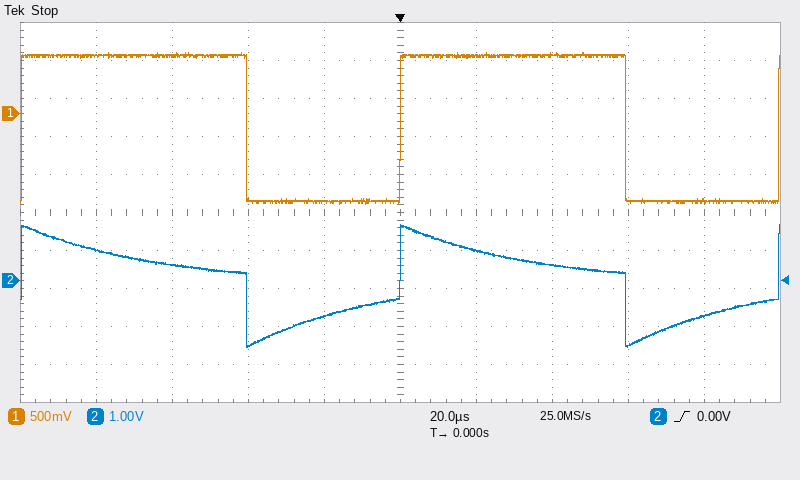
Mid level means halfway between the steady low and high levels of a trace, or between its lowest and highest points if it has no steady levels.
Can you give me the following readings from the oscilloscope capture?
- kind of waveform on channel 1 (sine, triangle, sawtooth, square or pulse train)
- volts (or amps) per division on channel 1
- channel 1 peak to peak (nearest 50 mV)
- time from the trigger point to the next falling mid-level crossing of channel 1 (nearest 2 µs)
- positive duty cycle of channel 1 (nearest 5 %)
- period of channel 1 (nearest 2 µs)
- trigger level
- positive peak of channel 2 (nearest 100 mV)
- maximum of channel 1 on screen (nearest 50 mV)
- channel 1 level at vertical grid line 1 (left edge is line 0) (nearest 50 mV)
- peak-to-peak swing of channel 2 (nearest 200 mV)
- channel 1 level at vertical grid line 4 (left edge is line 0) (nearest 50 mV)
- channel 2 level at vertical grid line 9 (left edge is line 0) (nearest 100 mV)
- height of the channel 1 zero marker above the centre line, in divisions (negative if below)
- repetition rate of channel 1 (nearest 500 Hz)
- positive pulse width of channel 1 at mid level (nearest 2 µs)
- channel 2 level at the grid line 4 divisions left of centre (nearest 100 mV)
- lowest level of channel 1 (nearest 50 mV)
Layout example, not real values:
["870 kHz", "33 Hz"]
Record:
["pulse train", "500 mV", "2.00 V", "60 µs", "60 %", "100 µs", "0.00 V", "1.5 V", "800 mV", "750 mV", "3.2 V", "-1.15 V", "-900 mV", "+2.6 div", "10.0 kHz", "60 µs", "800 mV", "-1.20 V"]
